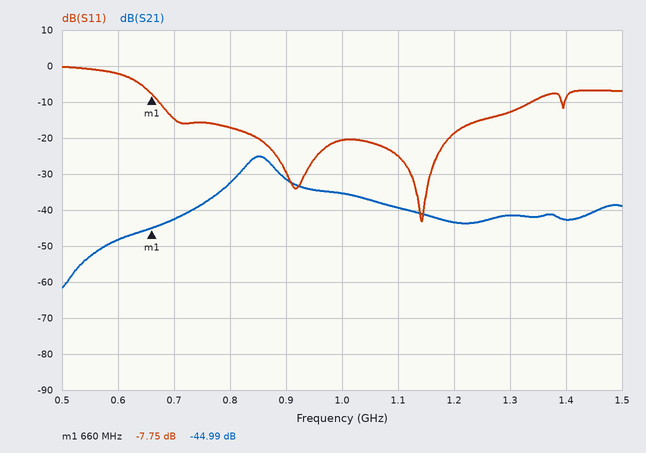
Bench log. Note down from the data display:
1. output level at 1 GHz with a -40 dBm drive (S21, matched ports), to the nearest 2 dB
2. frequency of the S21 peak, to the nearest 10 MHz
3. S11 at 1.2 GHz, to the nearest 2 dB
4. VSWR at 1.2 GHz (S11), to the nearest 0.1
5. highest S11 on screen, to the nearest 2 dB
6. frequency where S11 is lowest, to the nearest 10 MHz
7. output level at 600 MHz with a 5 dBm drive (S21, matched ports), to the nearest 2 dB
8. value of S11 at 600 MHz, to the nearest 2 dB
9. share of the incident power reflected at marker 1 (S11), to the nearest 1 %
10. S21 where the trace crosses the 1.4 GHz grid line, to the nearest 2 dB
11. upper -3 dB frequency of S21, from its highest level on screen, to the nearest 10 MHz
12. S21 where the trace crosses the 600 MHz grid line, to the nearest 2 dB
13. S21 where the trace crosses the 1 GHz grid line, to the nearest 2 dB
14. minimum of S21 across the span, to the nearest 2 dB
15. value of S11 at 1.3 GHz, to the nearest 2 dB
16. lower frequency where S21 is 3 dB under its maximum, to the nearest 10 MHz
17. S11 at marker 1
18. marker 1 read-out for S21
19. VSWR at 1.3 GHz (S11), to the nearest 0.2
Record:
-76 dBm
850 MHz
-18 dB
1.3
0 dB
1.14 GHz
-44 dBm
-2 dB
17 %
-42 dB
880 MHz
-48 dB
-36 dB
-62 dB
-12 dB
830 MHz
-7.75 dB
-44.99 dB
1.6
